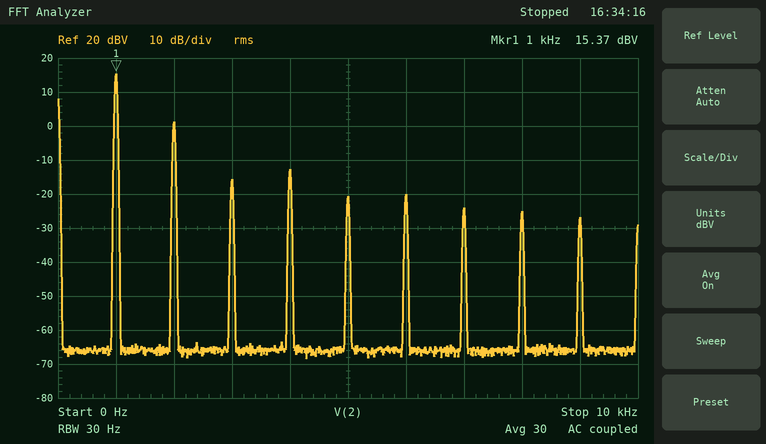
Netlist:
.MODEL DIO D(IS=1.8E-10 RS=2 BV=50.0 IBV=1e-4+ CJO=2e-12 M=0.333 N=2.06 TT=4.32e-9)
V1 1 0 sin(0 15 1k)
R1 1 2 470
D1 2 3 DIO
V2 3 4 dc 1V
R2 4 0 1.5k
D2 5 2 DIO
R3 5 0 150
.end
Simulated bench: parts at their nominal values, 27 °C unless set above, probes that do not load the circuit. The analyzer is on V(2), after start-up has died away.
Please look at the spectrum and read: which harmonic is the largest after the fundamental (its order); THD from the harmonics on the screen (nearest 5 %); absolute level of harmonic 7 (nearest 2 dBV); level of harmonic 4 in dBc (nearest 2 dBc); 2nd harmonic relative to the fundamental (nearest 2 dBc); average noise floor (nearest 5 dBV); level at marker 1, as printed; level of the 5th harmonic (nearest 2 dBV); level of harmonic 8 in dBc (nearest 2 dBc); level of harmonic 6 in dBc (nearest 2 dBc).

2
20 %
-24 dBV
-28 dBc
-14 dBc
-65 dBV
15.37 dBV
-20 dBV
-40 dBc
-36 dBc
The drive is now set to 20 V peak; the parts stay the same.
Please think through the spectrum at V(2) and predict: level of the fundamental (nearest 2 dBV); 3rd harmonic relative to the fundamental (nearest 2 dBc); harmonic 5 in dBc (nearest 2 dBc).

18 dBV
-34 dBc
-38 dBc
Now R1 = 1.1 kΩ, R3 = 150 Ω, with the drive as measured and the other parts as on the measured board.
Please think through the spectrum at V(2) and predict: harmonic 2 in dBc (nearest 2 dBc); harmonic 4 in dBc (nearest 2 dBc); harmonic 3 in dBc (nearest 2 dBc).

-12 dBc
-26 dBc
-26 dBc
